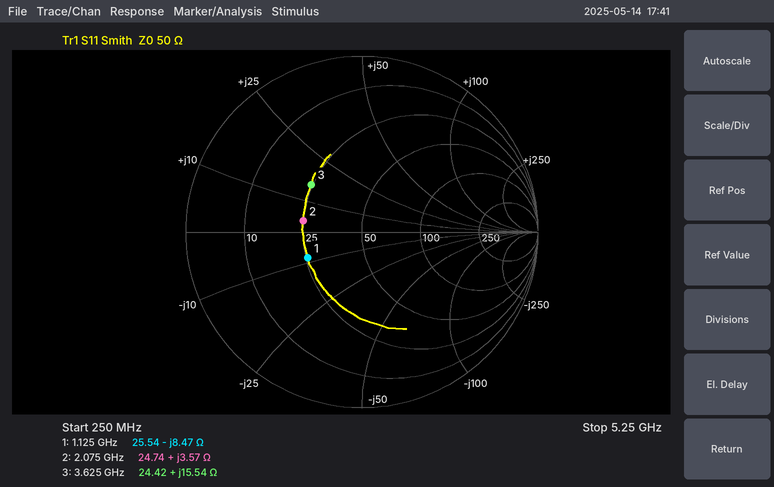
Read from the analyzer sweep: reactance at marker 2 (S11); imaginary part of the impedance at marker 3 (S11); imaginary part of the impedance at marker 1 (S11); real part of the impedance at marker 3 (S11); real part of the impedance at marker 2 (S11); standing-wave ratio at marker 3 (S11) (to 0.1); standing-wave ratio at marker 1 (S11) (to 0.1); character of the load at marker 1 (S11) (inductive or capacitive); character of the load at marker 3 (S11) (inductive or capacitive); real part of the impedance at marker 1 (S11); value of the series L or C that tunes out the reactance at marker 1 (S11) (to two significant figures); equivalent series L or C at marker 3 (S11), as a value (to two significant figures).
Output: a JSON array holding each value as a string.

["+3.57 Ω", "+15.54 Ω", "-8.47 Ω", "24.42 Ω", "24.74 Ω", "2.3", "2.0", "capacitive", "inductive", "25.54 Ω", "1.2 nH", "680 pH"]
